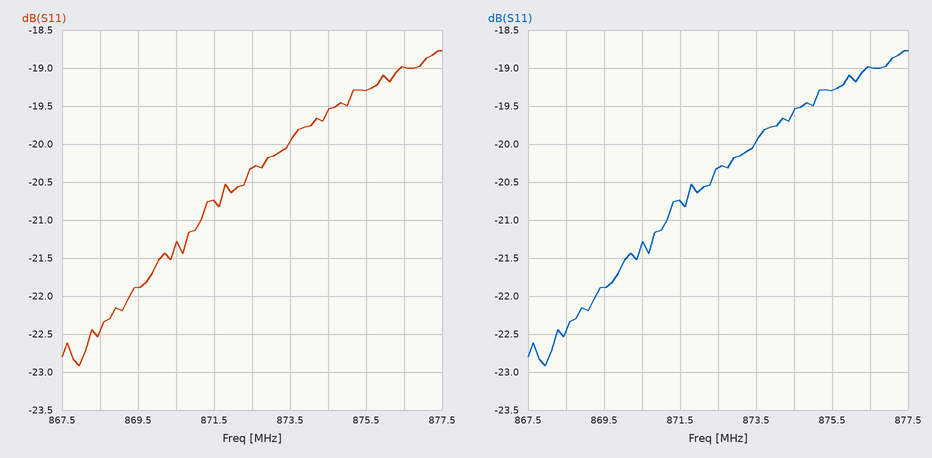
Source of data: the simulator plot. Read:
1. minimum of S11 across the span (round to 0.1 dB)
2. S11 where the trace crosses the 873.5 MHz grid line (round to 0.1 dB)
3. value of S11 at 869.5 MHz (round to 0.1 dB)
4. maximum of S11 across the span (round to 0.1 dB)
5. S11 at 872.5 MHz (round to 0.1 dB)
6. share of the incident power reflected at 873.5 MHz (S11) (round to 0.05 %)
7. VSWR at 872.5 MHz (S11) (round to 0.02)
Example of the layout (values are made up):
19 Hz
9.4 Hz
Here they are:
-22.9 dB
-20.0 dB
-21.9 dB
-18.8 dB
-20.3 dB
1.00 %
1.22
